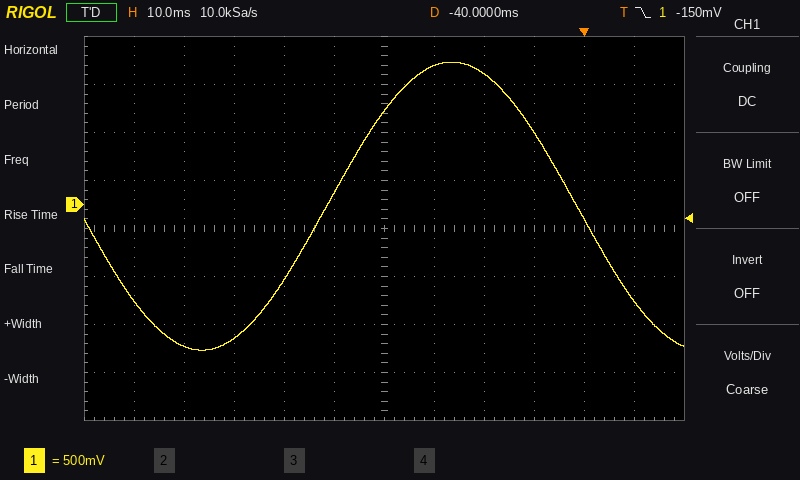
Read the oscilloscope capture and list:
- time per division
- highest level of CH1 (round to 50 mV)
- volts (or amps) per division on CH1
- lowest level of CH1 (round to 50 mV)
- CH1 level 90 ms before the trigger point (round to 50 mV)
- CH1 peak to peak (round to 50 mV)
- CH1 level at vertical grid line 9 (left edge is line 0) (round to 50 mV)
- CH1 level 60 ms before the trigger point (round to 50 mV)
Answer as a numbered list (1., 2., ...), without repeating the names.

1. 10 ms
2. 1.50 V
3. 500 mV
4. -1.50 V
5. -1.00 V
6. 3.00 V
7. 750 mV
8. -800 mV
